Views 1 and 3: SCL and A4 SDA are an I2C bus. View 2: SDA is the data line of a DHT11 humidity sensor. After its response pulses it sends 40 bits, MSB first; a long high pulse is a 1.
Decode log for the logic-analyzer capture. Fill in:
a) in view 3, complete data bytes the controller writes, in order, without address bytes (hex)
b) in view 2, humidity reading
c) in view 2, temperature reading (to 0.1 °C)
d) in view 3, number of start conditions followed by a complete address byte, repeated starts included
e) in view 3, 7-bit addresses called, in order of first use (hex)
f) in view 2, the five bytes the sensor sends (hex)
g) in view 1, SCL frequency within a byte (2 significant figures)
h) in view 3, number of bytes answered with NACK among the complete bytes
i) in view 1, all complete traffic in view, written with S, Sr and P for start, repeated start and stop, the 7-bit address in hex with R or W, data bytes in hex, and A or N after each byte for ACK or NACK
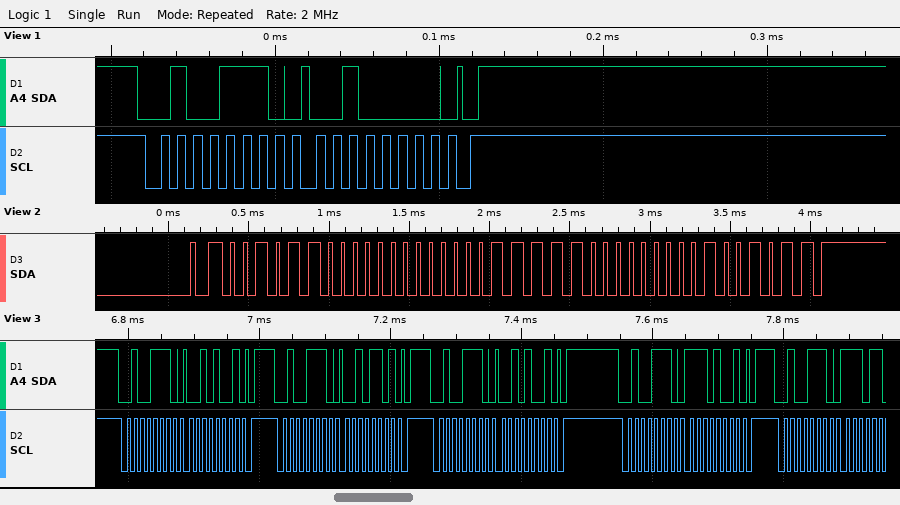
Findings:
29 2D 29 E9
44 %
31.0 °C
5
0x27
2C 00 1F 00 4B
100 kHz
0
S 27W A 20 A P
